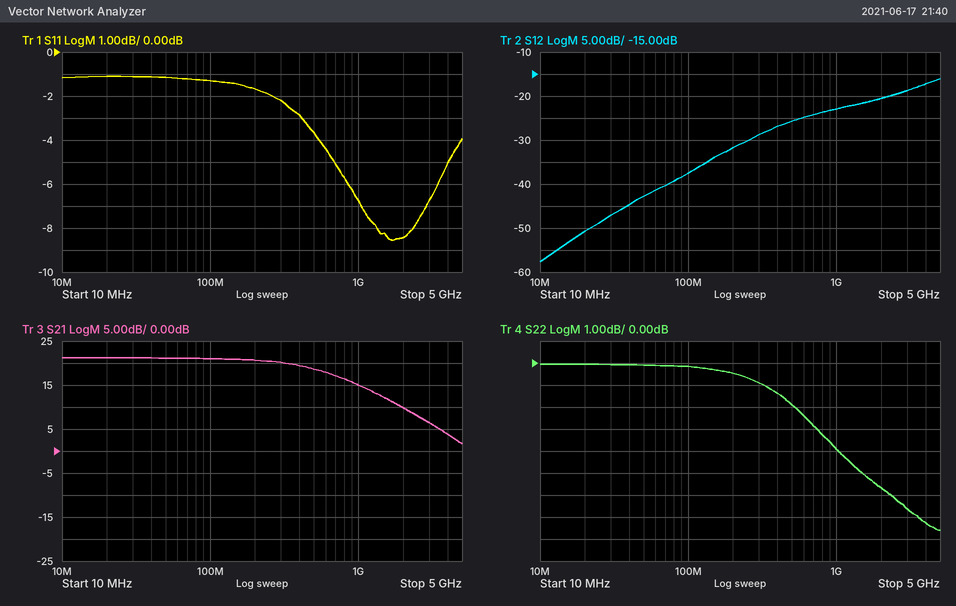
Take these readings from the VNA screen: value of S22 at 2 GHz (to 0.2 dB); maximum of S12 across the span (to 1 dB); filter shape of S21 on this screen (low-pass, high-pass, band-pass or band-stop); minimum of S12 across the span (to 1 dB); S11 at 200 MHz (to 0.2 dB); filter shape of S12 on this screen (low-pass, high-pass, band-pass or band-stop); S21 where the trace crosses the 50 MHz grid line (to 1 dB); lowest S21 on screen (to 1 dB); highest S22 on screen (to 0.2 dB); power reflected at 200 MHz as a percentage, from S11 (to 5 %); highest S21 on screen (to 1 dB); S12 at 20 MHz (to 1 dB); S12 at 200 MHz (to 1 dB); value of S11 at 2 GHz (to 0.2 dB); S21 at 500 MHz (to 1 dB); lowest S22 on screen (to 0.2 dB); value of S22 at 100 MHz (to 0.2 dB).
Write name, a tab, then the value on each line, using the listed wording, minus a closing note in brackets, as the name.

value of S22 at 2 GHz	-5.6 dB
maximum of S12 across the span	-16 dB
filter shape of S21 on this screen	low-pass
minimum of S12 across the span	-58 dB
S11 at 200 MHz	-1.6 dB
filter shape of S12 on this screen	high-pass
S21 where the trace crosses the 50 MHz grid line	21 dB
lowest S21 on screen	2 dB
highest S22 on screen	0.0 dB
power reflected at 200 MHz as a percentage, from S11	70 %
highest S21 on screen	21 dB
S12 at 20 MHz	-51 dB
S12 at 200 MHz	-32 dB
value of S11 at 2 GHz	-8.4 dB
S21 at 500 MHz	19 dB
lowest S22 on screen	-7.6 dB
value of S22 at 100 MHz	-0.2 dB
